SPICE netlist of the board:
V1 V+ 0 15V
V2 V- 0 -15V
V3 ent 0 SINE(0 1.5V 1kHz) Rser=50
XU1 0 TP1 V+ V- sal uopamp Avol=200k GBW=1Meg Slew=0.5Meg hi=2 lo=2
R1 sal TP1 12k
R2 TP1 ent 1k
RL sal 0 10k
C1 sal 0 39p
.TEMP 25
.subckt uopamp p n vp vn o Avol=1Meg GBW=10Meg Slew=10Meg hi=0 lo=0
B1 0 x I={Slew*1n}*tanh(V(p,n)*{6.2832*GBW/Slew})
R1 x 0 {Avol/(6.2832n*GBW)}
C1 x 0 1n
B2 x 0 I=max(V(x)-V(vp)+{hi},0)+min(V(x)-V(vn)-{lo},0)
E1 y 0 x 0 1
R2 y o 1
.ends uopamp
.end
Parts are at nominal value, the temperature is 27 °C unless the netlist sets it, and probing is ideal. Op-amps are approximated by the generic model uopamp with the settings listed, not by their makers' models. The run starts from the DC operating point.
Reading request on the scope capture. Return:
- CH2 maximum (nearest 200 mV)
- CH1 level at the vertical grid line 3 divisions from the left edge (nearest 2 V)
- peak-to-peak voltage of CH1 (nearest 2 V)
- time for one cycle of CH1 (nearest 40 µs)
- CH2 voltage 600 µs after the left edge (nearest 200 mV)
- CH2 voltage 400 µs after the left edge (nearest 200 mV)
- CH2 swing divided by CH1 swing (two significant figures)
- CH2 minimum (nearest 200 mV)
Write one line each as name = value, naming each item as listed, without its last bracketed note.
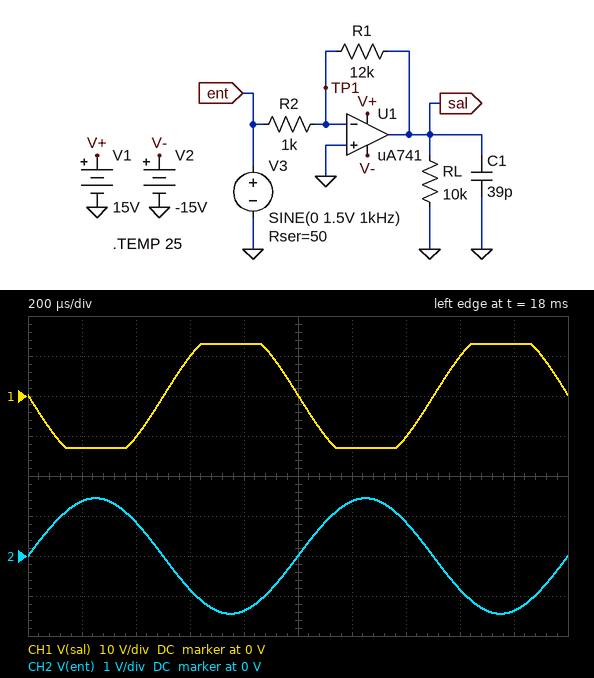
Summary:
CH2 maximum = 1.4 V
CH1 level at the vertical grid line 3 divisions from the left edge = 10 V
peak-to-peak voltage of CH1 = 26 V
time for one cycle of CH1 = 1.00 ms
CH2 voltage 600 µs after the left edge = -800 mV
CH2 voltage 400 µs after the left edge = 800 mV
CH2 swing divided by CH1 swing = 0.11
CH2 minimum = -1.4 V
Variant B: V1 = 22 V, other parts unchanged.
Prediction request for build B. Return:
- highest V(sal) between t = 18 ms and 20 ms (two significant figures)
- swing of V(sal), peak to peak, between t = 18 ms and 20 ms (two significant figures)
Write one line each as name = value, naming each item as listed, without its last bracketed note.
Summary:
highest V(sal) between t = 18 ms and 20 ms = 17 V
swing of V(sal), peak to peak, between t = 18 ms and 20 ms = 30 V
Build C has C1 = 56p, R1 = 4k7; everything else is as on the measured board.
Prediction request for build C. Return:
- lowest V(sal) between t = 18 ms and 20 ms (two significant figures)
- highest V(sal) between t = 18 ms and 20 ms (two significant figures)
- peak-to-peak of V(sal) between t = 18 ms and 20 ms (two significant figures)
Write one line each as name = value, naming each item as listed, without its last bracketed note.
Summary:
lowest V(sal) between t = 18 ms and 20 ms = -6.7 V
highest V(sal) between t = 18 ms and 20 ms = 6.7 V
peak-to-peak of V(sal) between t = 18 ms and 20 ms = 13 V
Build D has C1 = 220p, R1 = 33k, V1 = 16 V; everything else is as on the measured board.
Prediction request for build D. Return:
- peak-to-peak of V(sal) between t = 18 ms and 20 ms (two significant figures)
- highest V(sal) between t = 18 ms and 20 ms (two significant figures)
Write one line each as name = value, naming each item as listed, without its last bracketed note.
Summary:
peak-to-peak of V(sal) between t = 18 ms and 20 ms = 27 V
highest V(sal) between t = 18 ms and 20 ms = 14 V
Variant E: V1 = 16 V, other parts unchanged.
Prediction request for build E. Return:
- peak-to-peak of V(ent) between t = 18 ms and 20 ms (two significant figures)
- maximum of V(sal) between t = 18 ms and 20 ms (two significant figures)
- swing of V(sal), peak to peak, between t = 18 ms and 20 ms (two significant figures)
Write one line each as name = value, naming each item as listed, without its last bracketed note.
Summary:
peak-to-peak of V(ent) between t = 18 ms and 20 ms = 2.9 V
maximum of V(sal) between t = 18 ms and 20 ms = 14 V
swing of V(sal), peak to peak, between t = 18 ms and 20 ms = 27 V
